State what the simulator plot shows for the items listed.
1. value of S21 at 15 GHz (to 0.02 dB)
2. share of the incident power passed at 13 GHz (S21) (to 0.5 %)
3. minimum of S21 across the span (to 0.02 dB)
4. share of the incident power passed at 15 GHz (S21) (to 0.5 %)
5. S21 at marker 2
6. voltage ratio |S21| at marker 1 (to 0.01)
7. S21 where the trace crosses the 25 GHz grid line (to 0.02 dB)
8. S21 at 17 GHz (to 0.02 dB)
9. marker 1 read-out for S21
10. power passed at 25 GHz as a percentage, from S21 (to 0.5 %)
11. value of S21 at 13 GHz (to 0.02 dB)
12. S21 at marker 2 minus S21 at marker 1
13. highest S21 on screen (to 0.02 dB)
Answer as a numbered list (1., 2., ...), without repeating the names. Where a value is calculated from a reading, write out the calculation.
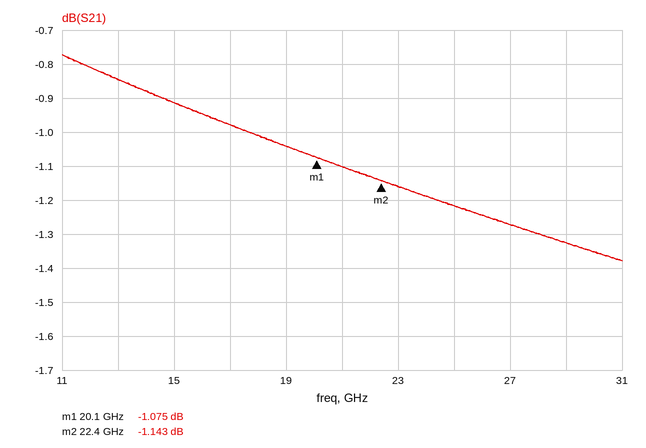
1. -0.92 dB
2. 10^(-0.84/10) ≈ 82.4 %, so 82.5 % to the nearest 0.5 %
3. -1.38 dB
4. 10^(-0.92/10) ≈ 80.9 %, so 81.0 % to the nearest 0.5 %
5. -1.143 dB
6. 10^(-1.075/20) ≈ 0.88
7. -1.22 dB
8. -0.98 dB
9. -1.075 dB
10. 10^(-1.22/10) ≈ 75.5 %
11. -0.84 dB
12. -1.143 − (-1.075) = -0.068 dB
13. -0.78 dB
